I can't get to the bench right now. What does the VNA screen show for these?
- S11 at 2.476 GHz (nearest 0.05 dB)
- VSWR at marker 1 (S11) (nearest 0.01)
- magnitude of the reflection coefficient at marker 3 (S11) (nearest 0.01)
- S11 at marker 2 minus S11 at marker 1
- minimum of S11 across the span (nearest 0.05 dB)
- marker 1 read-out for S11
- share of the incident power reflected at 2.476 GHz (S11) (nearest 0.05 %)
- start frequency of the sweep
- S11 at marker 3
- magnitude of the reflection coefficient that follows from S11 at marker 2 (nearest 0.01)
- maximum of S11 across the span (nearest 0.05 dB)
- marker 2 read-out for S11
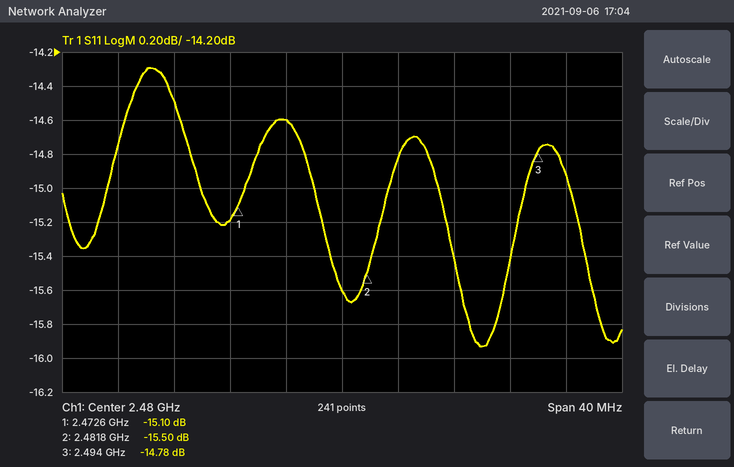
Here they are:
-14.60 dB
1.43
0.18
-0.40 dB
-15.95 dB
-15.10 dB
3.45 %
2.46 GHz
-14.78 dB
0.17
-14.30 dB
-15.50 dB
